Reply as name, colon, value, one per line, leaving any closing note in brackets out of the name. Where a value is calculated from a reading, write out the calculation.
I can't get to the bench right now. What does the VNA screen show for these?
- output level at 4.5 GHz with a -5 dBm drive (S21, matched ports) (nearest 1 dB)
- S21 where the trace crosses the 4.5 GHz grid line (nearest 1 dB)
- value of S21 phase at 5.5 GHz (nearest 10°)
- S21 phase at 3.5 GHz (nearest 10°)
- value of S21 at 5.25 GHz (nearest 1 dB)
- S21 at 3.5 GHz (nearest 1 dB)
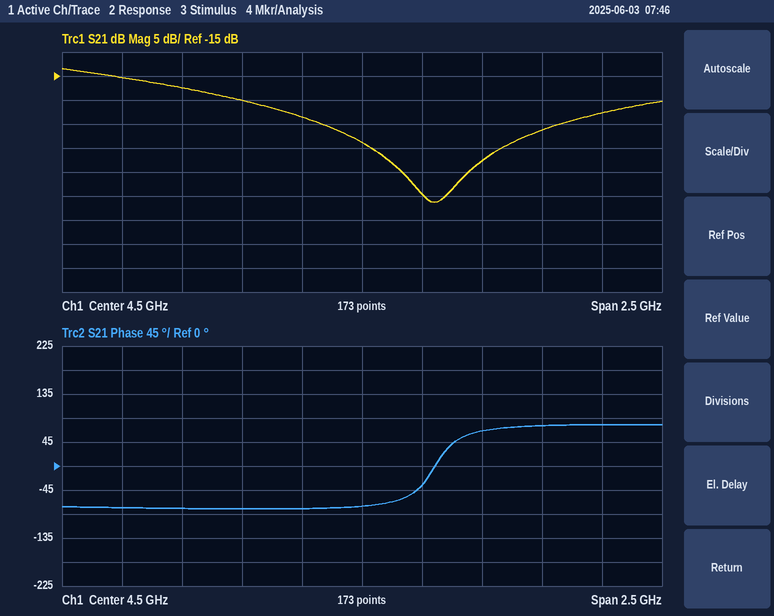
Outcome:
output level at 4.5 GHz with a -5 dBm drive (S21, matched ports): -5 dBm + (-29 dB) = -34 dBm
S21 where the trace crosses the 4.5 GHz grid line: -29 dB
value of S21 phase at 5.5 GHz: 80°
S21 phase at 3.5 GHz: -80°
value of S21 at 5.25 GHz: -26 dB
S21 at 3.5 GHz: -15 dB
